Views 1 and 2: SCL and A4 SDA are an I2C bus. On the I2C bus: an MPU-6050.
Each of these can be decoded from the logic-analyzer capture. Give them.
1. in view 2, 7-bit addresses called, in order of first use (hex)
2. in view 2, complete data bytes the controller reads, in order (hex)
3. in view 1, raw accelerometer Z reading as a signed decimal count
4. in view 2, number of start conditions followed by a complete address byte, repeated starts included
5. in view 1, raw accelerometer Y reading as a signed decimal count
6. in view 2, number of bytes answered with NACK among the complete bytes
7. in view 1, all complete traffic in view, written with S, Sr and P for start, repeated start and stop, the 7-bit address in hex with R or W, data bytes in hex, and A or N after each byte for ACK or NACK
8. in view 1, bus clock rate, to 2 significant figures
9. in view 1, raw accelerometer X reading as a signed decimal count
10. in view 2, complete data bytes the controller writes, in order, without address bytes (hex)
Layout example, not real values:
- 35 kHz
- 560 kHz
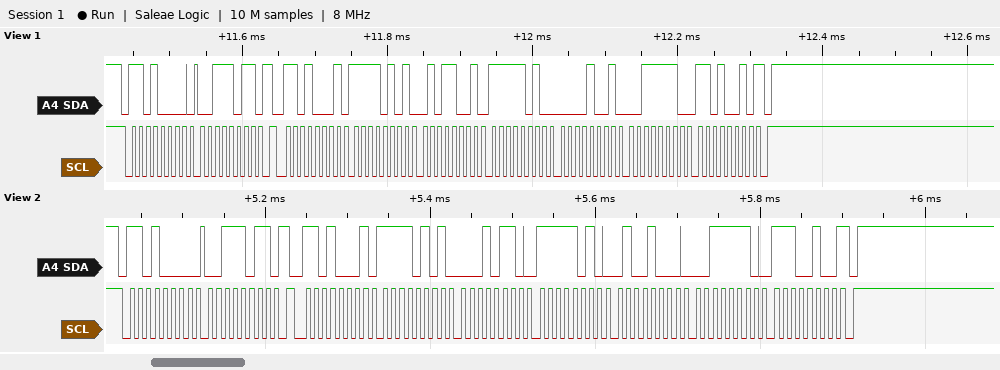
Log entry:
- 0x68
- F5 16 FA 48 3E E4
- 16082
- 2
- -1527
- 1
- S 68W A 3B A Sr 68R A F5 A 59 A FA A 09 A 3E A D2 N P
- 100 kHz
- -2727
- 3B
